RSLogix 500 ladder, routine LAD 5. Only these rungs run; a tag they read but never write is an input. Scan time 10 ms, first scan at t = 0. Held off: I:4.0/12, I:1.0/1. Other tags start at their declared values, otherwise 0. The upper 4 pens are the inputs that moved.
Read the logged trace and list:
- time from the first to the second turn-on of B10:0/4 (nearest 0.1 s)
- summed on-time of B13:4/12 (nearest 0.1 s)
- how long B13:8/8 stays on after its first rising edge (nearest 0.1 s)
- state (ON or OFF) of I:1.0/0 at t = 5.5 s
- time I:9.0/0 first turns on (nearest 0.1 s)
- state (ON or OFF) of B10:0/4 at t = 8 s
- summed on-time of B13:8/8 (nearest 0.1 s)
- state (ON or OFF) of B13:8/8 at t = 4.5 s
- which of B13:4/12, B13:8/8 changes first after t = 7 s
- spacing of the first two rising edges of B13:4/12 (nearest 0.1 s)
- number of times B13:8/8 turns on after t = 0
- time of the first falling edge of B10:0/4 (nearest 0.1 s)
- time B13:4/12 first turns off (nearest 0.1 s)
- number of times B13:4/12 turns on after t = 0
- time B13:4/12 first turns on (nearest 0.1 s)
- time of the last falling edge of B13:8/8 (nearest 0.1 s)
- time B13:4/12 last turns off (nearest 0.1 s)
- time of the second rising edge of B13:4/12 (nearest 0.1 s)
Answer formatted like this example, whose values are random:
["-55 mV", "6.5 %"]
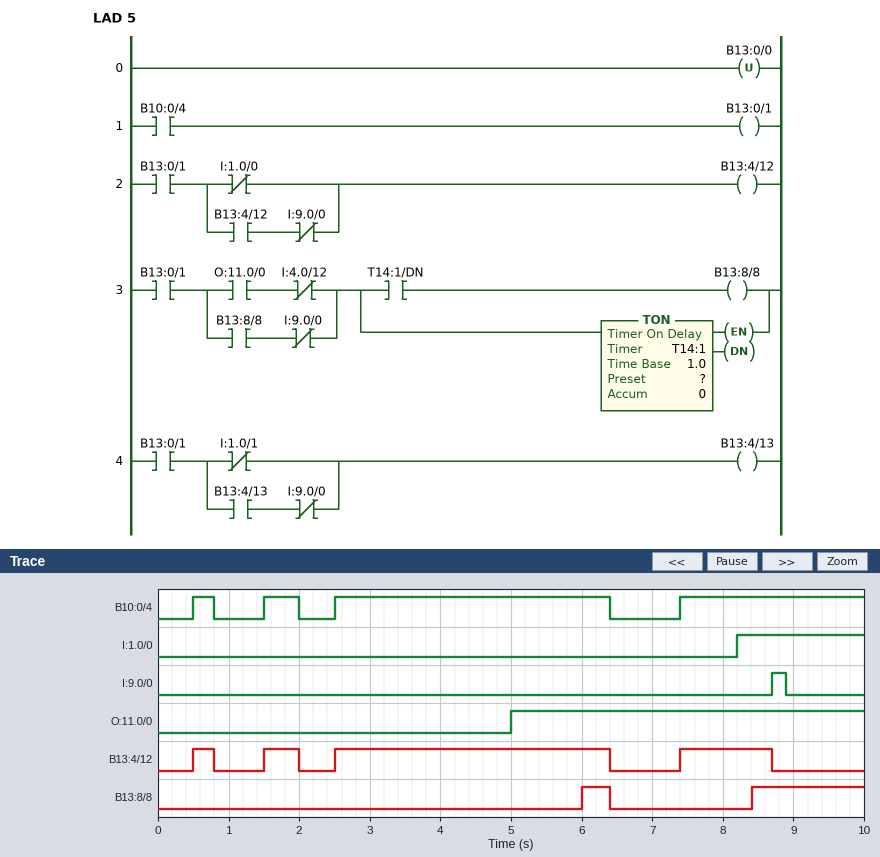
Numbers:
["1.0 s", "6.0 s", "0.4 s", "OFF", "8.7 s", "ON", "2.0 s", "OFF", "B13:4/12", "1.0 s", "2", "0.8 s", "0.8 s", "4", "0.5 s", "6.4 s", "8.7 s", "1.5 s"]
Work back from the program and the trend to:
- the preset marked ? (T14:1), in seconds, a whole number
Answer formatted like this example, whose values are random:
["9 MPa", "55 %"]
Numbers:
["1 s"]
